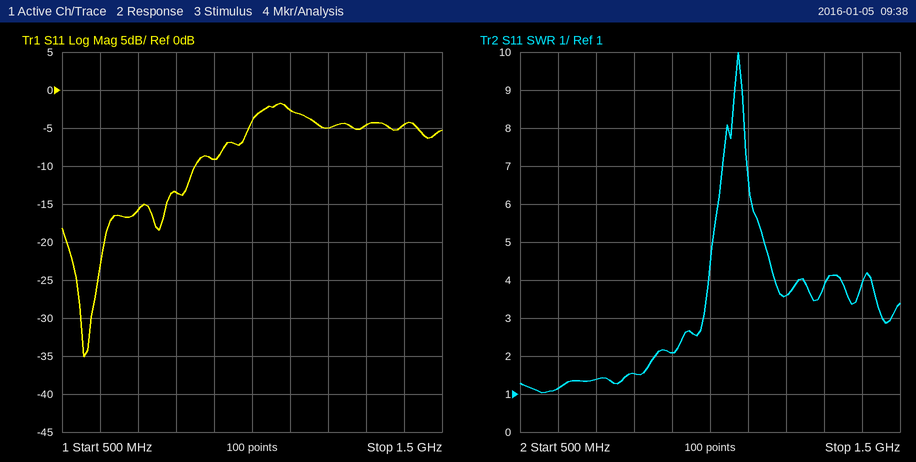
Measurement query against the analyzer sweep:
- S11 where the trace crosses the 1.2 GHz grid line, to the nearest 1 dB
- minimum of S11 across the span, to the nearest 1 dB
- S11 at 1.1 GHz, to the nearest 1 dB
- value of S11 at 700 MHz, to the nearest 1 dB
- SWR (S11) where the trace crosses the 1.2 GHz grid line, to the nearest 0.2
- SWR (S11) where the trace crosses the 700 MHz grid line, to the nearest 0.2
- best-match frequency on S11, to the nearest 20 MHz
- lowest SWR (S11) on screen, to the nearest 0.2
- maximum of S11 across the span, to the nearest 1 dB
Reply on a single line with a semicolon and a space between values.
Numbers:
-5 dB; -35 dB; -3 dB; -16 dB; 3.6; 1.4; 560 MHz; 1.0; -2 dB
